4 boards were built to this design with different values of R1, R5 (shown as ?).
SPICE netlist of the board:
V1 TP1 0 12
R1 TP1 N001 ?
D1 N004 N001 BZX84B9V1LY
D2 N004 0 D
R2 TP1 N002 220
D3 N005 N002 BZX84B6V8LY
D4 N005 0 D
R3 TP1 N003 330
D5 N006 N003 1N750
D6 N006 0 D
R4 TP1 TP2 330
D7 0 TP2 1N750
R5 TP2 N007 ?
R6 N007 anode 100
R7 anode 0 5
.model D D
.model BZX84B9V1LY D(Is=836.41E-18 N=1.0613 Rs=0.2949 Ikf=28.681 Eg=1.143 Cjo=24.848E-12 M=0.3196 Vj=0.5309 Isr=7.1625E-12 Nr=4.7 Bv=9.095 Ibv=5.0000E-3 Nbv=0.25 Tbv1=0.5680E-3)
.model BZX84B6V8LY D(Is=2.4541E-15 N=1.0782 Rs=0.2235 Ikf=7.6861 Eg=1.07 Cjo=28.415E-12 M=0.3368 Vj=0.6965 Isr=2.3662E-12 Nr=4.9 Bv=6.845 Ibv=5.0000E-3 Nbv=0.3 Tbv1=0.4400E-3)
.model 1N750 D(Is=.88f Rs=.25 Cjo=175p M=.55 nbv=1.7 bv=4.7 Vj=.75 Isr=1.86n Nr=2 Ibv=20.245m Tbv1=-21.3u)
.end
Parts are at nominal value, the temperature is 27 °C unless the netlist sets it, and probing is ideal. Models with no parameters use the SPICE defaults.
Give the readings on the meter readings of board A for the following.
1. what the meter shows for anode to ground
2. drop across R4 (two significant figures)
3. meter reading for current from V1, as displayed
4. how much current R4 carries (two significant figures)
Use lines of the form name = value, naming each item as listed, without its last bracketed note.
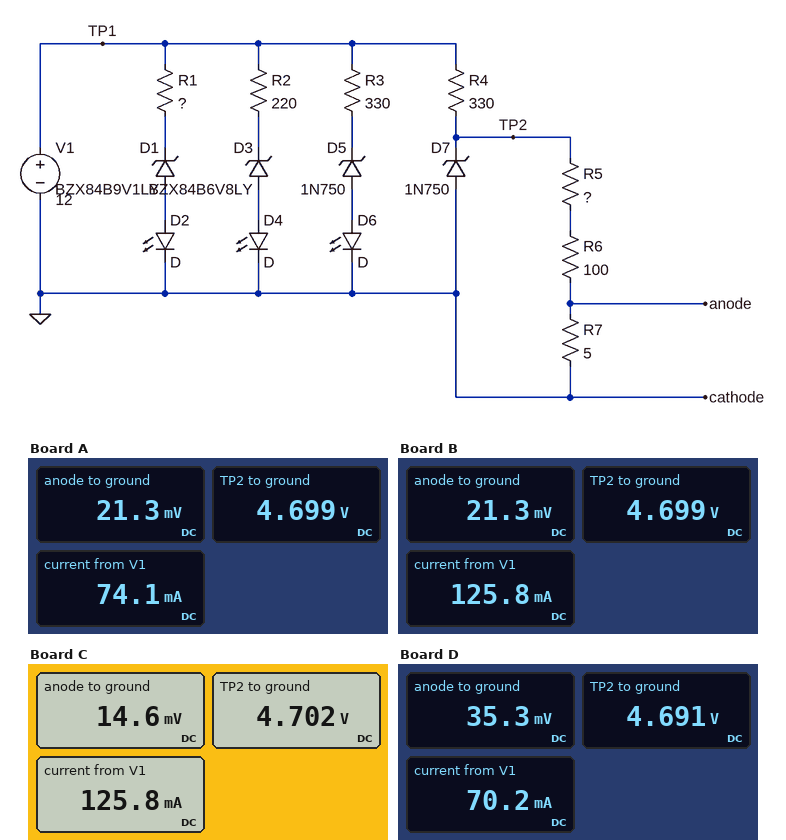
what the meter shows for anode to ground = 21.3 mV
drop across R4 = 7.3 V
meter reading for current from V1, as displayed = 74.1 mA
how much current R4 carries = 22 mA
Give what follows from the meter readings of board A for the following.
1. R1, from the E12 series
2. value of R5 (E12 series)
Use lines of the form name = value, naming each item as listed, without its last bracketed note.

R1, from the E12 series = 180 Ω
value of R5 = 1 kΩ
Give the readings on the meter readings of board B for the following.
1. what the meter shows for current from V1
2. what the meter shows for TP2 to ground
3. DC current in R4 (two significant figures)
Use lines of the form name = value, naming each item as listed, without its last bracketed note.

what the meter shows for current from V1 = 125.8 mA
what the meter shows for TP2 to ground = 4.699 V
DC current in R4 = 22 mA
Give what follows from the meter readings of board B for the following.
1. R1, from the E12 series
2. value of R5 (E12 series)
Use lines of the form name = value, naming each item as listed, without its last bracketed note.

R1, from the E12 series = 33 Ω
value of R5 = 1 kΩ
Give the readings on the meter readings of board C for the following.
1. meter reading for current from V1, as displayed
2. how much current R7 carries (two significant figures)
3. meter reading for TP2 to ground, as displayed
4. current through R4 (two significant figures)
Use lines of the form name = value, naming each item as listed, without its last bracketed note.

meter reading for current from V1, as displayed = 125.8 mA
how much current R7 carries = 2.9 mA
meter reading for TP2 to ground, as displayed = 4.702 V
current through R4 = 22 mA
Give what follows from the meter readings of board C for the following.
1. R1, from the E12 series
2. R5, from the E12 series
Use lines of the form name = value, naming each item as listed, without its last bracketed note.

R1, from the E12 series = 33 Ω
R5, from the E12 series = 1.5 kΩ
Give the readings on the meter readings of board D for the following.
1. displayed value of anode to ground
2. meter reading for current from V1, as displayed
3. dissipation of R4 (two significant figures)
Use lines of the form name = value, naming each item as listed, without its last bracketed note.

displayed value of anode to ground = 35.3 mV
meter reading for current from V1, as displayed = 70.2 mA
dissipation of R4 = 160 mW
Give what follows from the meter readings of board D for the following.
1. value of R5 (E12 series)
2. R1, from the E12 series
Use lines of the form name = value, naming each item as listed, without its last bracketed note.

value of R5 = 560 Ω
R1, from the E12 series = 270 Ω
